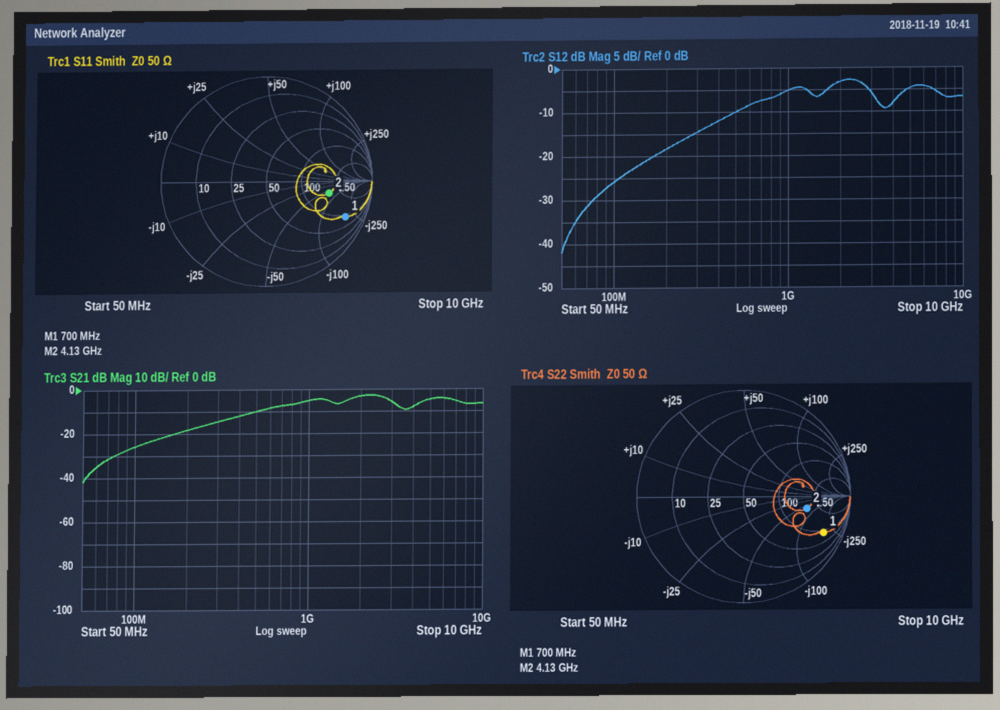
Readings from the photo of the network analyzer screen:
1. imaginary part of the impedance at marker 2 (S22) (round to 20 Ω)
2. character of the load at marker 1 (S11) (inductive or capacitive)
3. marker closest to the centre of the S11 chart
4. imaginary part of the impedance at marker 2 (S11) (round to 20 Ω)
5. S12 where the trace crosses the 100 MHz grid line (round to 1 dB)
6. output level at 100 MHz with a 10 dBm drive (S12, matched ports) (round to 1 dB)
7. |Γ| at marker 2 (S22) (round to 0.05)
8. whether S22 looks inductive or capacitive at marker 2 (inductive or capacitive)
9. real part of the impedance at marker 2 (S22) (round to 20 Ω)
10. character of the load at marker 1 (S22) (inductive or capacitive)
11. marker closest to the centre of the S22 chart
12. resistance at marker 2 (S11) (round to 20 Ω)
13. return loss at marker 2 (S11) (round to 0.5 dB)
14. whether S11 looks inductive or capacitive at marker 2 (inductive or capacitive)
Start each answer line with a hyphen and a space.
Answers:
- -60 Ω
- capacitive
- marker 2
- -60 Ω
- -26 dB
- -16 dBm
- 0.60
- capacitive
- 180 Ω
- capacitive
- marker 2
- 180 Ω
- 4.5 dB
- capacitive
